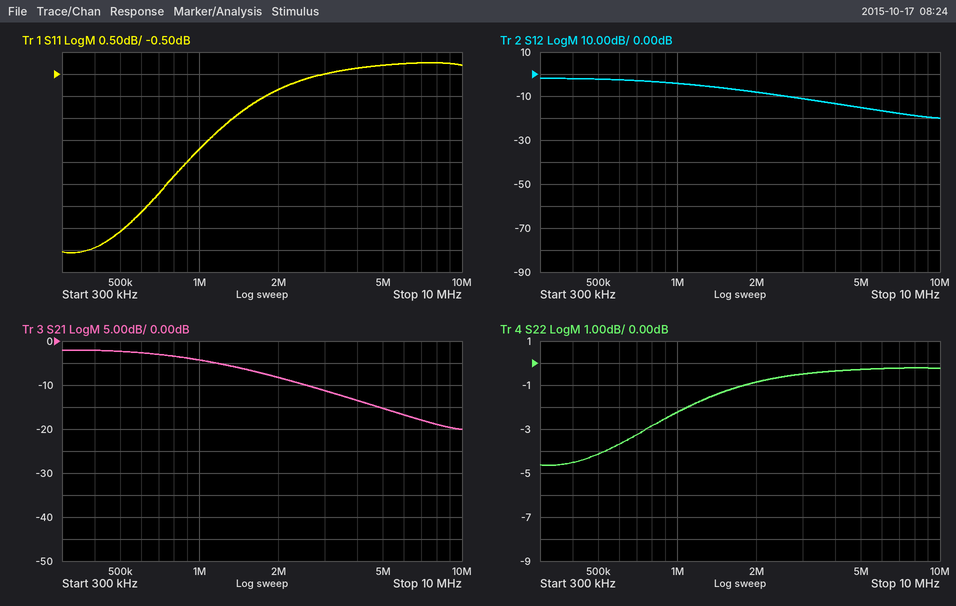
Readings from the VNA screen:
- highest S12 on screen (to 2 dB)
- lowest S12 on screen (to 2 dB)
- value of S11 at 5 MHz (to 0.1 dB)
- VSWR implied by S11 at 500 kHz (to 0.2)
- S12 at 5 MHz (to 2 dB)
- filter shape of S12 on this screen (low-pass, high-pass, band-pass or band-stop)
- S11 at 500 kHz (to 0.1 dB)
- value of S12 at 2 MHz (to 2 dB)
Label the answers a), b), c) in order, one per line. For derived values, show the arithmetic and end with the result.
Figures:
a) -2 dB
b) -20 dB
c) -0.3 dB
d) |Γ| = 10^(-4.1/20) = 0.6237; VSWR = (1 + 0.6237)/(1 − 0.6237) ≈ 4.32, so 4.4 to the nearest 0.2
e) -16 dB
f) low-pass
g) -4.1 dB
h) -8 dB
